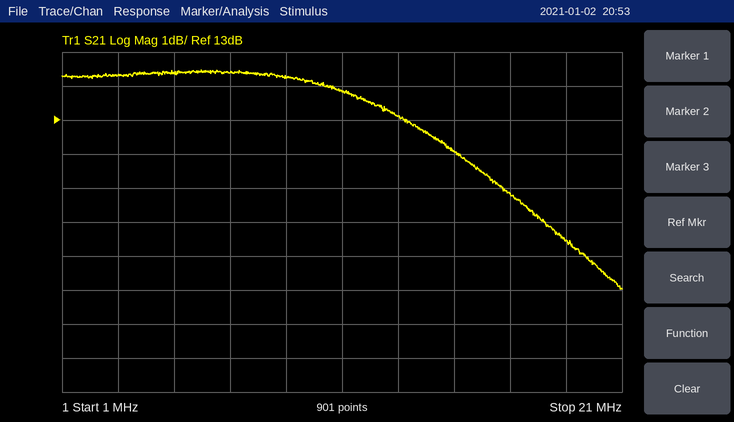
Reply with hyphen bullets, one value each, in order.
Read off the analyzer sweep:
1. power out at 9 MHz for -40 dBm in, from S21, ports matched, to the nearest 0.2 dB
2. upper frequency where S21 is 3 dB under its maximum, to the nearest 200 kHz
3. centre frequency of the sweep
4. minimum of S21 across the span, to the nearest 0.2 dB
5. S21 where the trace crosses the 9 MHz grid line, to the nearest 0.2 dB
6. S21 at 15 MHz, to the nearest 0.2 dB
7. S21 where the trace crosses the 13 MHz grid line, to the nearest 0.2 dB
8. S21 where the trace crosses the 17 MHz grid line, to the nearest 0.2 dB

- -25.8 dBm
- 16.0 MHz
- 11 MHz
- 8.0 dB
- 14.2 dB
- 12.0 dB
- 13.2 dB
- 10.8 dB
